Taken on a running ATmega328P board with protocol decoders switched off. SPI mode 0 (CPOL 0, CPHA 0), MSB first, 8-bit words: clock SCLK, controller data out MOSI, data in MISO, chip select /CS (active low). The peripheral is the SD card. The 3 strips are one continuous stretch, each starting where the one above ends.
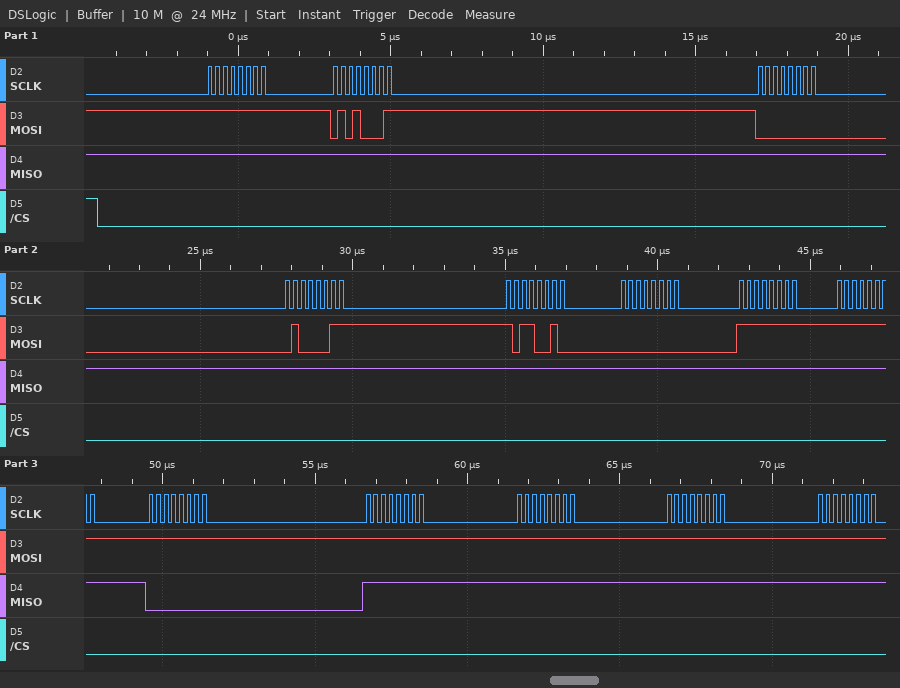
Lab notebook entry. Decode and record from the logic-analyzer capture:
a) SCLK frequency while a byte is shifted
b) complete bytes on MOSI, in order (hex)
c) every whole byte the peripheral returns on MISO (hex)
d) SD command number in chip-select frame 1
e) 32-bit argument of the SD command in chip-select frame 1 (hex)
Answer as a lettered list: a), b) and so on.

a) 4 MHz
b) 0xFF 0x51 0x00 0x43 0xB2 0x00 0xFF 0xFF 0xFF 0xFF 0xFF 0xFF 0xFF
c) 0xFF 0xFF 0xFF 0xFF 0xFF 0xFF 0xFF 0xFF 0x00 0xFF 0xFF 0xFF 0xFF
d) CMD17
e) 0x0043B200
